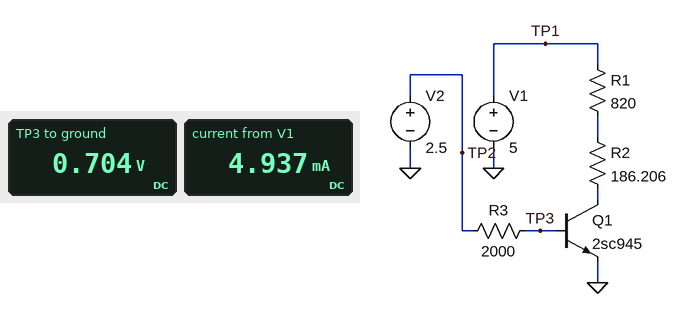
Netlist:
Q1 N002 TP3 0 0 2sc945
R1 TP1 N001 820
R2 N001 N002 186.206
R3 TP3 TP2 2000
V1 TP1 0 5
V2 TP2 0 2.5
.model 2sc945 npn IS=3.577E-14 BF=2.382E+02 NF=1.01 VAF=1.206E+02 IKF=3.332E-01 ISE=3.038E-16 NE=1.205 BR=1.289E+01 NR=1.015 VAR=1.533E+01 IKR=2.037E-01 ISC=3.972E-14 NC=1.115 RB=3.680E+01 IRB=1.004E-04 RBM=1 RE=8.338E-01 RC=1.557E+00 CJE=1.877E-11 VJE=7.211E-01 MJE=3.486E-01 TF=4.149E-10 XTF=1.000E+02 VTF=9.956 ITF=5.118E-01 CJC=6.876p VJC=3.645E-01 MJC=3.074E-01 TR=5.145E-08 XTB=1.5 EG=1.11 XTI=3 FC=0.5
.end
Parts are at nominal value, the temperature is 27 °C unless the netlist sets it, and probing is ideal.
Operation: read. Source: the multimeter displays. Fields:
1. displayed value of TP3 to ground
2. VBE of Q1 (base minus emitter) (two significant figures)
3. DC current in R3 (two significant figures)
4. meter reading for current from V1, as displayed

0.704 V
700 mV
900 µA
4.937 mA
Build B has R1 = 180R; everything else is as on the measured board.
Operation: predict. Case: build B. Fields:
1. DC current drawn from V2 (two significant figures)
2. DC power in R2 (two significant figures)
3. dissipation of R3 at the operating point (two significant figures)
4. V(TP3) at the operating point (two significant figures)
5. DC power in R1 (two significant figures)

890 µA
34 mW
1.6 mW
730 mV
33 mW
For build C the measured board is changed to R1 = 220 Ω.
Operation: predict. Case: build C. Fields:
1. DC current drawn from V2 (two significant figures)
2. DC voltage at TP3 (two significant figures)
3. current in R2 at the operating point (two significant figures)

890 µA
720 mV
12 mA
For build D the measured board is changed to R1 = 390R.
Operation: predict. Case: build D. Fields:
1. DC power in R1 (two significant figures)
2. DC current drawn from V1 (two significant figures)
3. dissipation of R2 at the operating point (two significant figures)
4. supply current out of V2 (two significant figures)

29 mW
8.6 mA
14 mW
890 µA
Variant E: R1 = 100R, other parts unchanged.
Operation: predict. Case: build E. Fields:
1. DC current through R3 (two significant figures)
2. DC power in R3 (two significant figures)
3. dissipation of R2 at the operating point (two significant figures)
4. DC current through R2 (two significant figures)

880 µA
1.6 mW
55 mW
17 mA
